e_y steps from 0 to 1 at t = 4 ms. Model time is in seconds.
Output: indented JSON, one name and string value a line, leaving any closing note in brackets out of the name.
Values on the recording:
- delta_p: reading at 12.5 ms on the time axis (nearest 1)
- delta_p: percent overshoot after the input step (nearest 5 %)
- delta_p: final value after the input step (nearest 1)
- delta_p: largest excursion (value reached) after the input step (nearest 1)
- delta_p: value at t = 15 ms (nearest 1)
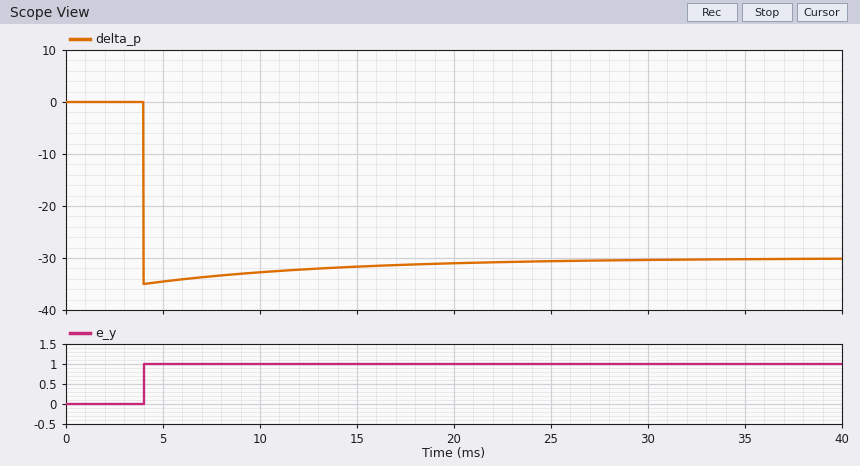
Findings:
{
  "delta_p: reading at 12.5 ms on the time axis": "-32",
  "delta_p: percent overshoot after the input step": "15 %",
  "delta_p: final value after the input step": "-30",
  "delta_p: largest excursion (value reached) after the input step": "-35",
  "delta_p: value at t = 15 ms": "-32"
}
